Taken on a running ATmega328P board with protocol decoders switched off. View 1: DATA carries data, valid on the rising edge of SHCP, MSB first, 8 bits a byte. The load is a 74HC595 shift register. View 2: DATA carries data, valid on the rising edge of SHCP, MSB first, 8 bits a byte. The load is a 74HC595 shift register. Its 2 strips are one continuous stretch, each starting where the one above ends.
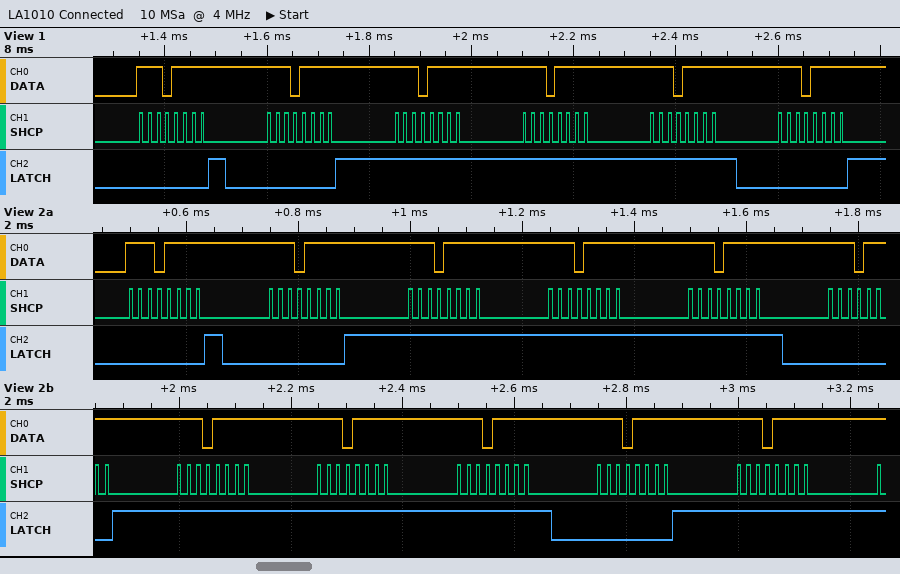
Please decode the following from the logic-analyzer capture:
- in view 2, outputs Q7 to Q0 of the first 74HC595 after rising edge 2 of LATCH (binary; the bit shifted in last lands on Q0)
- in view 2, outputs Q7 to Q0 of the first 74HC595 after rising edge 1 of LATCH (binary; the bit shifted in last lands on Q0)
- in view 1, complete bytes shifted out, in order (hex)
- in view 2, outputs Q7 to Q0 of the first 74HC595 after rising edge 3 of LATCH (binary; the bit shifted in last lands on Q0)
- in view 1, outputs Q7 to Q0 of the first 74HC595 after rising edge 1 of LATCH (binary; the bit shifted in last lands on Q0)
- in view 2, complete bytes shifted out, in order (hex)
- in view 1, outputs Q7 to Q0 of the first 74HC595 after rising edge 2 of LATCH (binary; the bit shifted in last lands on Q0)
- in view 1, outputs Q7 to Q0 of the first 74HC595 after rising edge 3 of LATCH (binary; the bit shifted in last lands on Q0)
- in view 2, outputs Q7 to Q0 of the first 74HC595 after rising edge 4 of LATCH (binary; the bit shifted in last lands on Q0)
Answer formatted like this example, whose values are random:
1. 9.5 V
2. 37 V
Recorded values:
1. 11101111
2. 11101111
3. 0xEF 0xEF 0xEF 0xEF 0xEF 0xEF
4. 11101111
5. 11101111
6. EF EF EF EF EF EF EF EF EF EF EF
7. 11101111
8. 11101111
9. 11101111
